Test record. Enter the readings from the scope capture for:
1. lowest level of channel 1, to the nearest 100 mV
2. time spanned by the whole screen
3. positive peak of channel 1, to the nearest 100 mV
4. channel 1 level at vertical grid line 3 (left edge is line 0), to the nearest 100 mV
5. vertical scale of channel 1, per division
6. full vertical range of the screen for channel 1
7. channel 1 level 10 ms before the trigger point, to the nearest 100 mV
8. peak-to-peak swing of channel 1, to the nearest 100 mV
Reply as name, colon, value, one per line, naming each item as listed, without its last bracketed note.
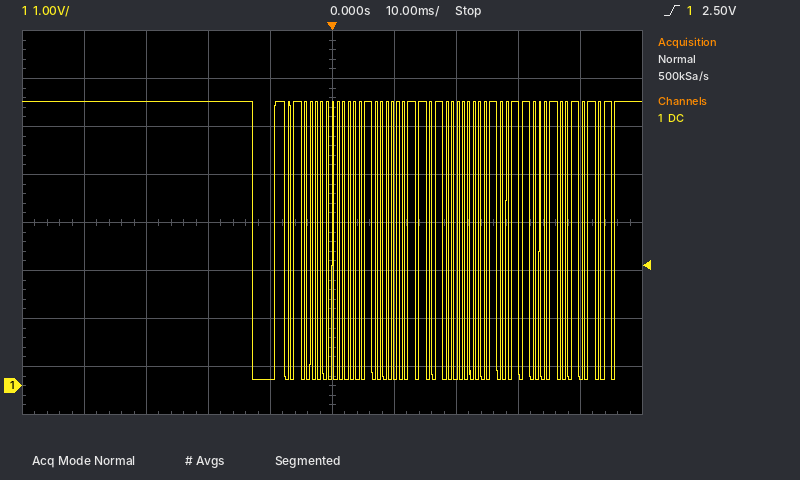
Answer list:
lowest level of channel 1, to the nearest 100 mV: 100 mV
time spanned by the whole screen: 100 ms
positive peak of channel 1, to the nearest 100 mV: 5.9 V
channel 1 level at vertical grid line 3 (left edge is line 0), to the nearest 100 mV: 5.9 V
vertical scale of channel 1, per division: 1 V
full vertical range of the screen for channel 1: 8 V
channel 1 level 10 ms before the trigger point, to the nearest 100 mV: 100 mV
peak-to-peak swing of channel 1, to the nearest 100 mV: 5.8 V
